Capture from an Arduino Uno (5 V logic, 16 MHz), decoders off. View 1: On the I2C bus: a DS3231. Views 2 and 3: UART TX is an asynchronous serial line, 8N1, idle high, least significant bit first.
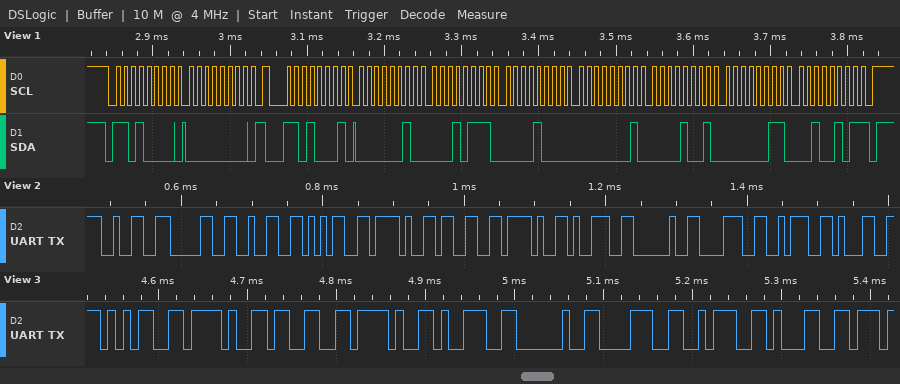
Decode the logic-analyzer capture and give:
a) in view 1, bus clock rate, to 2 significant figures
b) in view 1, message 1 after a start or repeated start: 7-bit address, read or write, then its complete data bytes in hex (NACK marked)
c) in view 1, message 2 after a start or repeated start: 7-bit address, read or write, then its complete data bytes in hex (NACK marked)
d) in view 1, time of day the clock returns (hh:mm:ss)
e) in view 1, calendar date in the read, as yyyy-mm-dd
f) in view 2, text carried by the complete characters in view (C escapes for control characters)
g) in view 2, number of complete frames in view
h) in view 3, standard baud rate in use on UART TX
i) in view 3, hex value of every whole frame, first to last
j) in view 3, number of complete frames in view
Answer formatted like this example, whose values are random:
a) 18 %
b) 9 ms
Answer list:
a) 100 kHz
b) 0x68 write: 00
c) 0x68 read: 02 17 08 01 09 03 25 NACK
d) 08:17:02
e) 2025-03-09
f) "2025/3/9 8:1"
g) 12
h) 115200 baud
i) 35 2F 33 2F 39 20 38 3A 31
j) 9
